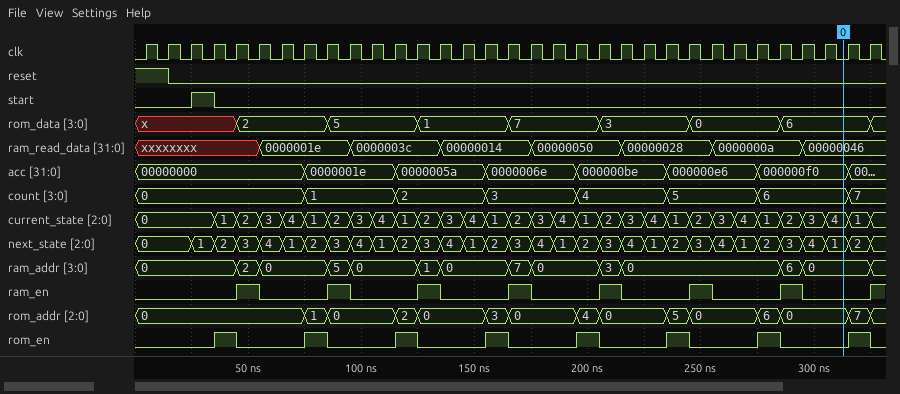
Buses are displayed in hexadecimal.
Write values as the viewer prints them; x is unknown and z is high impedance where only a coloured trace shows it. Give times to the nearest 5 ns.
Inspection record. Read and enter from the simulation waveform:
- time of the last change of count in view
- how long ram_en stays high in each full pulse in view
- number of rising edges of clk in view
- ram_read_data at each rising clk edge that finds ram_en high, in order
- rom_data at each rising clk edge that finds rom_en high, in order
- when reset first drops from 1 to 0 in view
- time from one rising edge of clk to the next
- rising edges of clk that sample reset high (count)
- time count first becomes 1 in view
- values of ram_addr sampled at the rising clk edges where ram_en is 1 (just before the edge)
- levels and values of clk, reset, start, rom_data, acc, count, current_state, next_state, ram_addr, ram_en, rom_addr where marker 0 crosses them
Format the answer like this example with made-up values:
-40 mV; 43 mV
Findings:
315 ns; 10 ns, 10 ns, 10 ns, 10 ns, 10 ns, 10 ns, 10 ns; 33; xxxxxxxx, 0000001e, 0000003c, 00000014, 00000050, 00000028, 0000000a; x, 2, 5, 1, 7, 3, 0, 6; 15 ns; 10 ns; 2; 75 ns; 2, 5, 1, 7, 3, 0, 6; clk=0, reset=0, start=0, rom_data=6, acc=000000f0, count=6, current_state=4, next_state=1, ram_addr=0, ram_en=0, rom_addr=0
